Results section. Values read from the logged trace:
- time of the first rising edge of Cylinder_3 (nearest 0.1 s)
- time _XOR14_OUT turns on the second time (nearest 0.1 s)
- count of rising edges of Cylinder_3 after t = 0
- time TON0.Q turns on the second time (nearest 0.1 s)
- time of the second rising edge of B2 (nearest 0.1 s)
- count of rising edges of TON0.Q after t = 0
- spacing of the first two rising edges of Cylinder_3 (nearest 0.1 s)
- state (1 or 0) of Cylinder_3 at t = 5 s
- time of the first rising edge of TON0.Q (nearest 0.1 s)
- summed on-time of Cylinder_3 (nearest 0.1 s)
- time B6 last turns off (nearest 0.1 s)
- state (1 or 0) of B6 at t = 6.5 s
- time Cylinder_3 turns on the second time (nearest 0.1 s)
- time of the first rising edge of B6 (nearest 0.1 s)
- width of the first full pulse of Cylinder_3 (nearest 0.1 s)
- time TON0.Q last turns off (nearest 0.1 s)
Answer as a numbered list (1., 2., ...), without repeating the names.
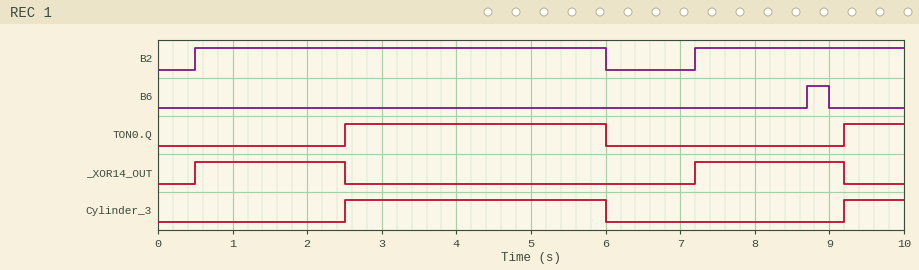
1. 2.5 s
2. 7.2 s
3. 2
4. 9.2 s
5. 7.2 s
6. 2
7. 6.7 s
8. 1
9. 2.5 s
10. 4.3 s
11. 9.0 s
12. 0
13. 9.2 s
14. 8.7 s
15. 3.5 s
16. 6.0 s
